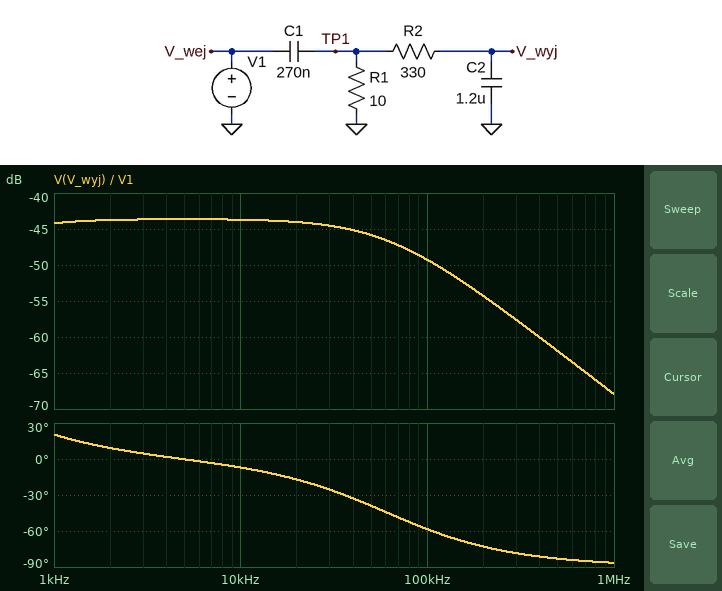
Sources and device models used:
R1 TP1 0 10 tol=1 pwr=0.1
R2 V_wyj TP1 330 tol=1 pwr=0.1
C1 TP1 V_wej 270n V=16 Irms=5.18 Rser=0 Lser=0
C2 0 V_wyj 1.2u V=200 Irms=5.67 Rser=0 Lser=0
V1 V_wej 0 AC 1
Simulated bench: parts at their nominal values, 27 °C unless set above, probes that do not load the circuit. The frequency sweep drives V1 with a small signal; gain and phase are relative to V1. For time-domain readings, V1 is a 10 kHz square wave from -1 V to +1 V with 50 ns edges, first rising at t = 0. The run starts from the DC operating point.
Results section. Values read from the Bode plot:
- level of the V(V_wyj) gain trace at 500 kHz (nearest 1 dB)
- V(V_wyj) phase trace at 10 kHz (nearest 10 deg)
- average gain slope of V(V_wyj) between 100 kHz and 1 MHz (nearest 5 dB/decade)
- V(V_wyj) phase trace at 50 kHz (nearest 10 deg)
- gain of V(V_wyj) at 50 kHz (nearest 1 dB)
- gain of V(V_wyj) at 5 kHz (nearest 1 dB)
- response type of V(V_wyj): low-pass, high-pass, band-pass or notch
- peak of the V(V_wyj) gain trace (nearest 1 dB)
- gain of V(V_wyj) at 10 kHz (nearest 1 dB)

-62 dB
-10 deg
-20 dB/decade
-40 deg
-46 dB
-44 dB
low-pass
-44 dB
-44 dB
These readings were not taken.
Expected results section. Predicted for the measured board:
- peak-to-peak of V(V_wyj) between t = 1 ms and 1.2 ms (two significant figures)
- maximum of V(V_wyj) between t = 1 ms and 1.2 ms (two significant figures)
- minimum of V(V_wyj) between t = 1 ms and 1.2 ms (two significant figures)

14 mV
7.3 mV
-6.4 mV
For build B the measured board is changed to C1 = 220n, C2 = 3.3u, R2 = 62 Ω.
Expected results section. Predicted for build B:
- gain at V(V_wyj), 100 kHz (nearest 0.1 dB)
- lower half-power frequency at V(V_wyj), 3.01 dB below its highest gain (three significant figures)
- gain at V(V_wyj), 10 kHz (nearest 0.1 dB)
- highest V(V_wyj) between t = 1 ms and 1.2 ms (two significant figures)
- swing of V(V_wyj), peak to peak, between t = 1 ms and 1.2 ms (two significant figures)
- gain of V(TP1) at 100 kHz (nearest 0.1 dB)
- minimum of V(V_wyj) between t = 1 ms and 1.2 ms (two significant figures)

-44.5 dB
659 Hz
-40.8 dB
9.9 mV
20 mV
-2.3 dB
-9.7 mV
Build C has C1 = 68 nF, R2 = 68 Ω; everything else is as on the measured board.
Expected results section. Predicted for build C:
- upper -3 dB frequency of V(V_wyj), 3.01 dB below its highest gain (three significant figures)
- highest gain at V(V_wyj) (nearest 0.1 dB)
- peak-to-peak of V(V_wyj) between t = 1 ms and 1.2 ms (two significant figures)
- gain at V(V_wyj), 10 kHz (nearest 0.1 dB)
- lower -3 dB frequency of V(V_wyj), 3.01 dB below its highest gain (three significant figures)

272 kHz
-42.8 dB
18 mV
-42.9 dB
1.68 kHz
